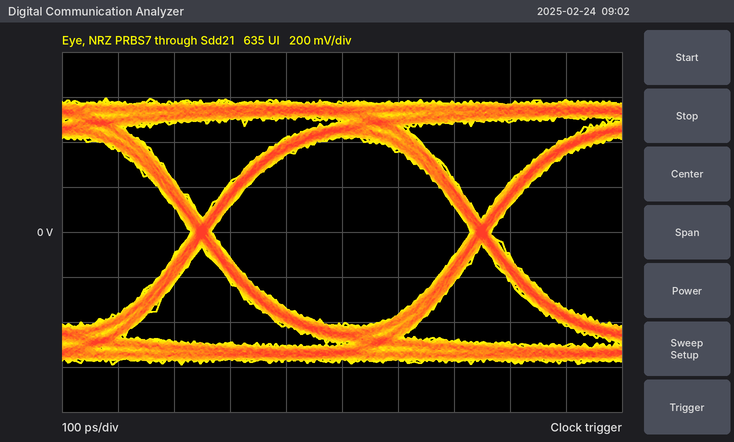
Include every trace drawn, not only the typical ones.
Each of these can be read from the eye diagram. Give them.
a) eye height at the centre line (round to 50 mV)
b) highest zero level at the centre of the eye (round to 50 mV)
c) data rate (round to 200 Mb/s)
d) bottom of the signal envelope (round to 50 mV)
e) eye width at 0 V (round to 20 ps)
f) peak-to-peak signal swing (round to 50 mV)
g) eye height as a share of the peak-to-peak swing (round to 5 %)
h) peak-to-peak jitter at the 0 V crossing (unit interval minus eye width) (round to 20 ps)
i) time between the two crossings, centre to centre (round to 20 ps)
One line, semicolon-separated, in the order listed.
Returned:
850 mV; -400 mV; 2.0 Gb/s; -600 mV; 460 ps; 1.20 V; 70 %; 40 ps; 500 ps
